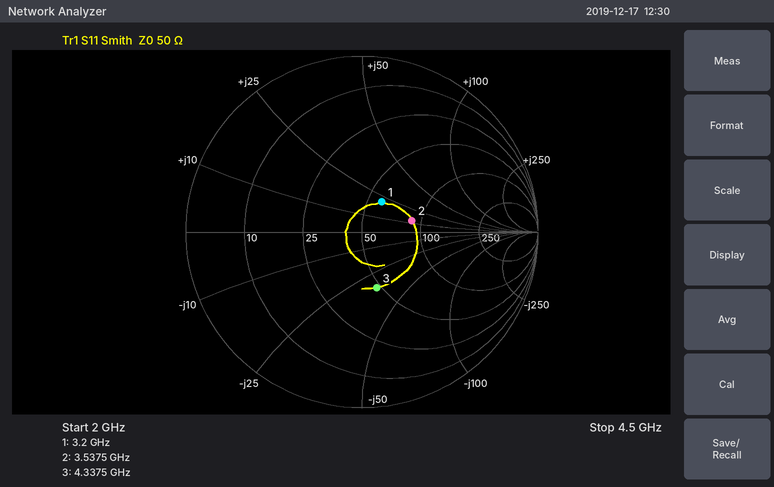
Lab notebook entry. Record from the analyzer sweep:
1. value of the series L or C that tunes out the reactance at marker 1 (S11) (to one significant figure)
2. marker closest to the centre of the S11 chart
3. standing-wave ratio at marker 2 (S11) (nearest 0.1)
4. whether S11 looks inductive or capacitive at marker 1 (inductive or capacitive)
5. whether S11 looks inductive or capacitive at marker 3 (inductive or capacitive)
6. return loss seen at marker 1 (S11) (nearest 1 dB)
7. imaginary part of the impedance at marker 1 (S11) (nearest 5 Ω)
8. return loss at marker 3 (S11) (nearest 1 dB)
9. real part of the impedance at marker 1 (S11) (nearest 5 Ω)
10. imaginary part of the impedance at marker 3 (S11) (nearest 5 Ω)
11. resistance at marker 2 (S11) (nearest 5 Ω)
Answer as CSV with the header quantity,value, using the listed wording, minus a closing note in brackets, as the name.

quantity,value
value of the series L or C that tunes out the reactance at marker 1 (S11),2 pF
marker closest to the centre of the S11 chart,marker 1
standing-wave ratio at marker 2 (S11),1.8
whether S11 looks inductive or capacitive at marker 1,inductive
whether S11 looks inductive or capacitive at marker 3,capacitive
return loss seen at marker 1 (S11),14 dB
imaginary part of the impedance at marker 1 (S11),+20 Ω
return loss at marker 3 (S11),10 dB
real part of the impedance at marker 1 (S11),60 Ω
imaginary part of the impedance at marker 3 (S11),-35 Ω
resistance at marker 2 (S11),90 Ω
